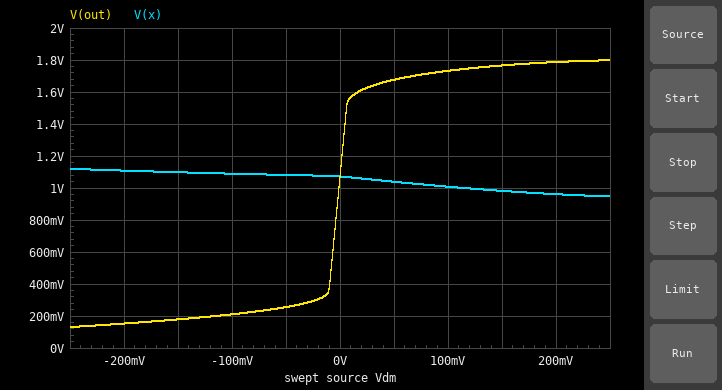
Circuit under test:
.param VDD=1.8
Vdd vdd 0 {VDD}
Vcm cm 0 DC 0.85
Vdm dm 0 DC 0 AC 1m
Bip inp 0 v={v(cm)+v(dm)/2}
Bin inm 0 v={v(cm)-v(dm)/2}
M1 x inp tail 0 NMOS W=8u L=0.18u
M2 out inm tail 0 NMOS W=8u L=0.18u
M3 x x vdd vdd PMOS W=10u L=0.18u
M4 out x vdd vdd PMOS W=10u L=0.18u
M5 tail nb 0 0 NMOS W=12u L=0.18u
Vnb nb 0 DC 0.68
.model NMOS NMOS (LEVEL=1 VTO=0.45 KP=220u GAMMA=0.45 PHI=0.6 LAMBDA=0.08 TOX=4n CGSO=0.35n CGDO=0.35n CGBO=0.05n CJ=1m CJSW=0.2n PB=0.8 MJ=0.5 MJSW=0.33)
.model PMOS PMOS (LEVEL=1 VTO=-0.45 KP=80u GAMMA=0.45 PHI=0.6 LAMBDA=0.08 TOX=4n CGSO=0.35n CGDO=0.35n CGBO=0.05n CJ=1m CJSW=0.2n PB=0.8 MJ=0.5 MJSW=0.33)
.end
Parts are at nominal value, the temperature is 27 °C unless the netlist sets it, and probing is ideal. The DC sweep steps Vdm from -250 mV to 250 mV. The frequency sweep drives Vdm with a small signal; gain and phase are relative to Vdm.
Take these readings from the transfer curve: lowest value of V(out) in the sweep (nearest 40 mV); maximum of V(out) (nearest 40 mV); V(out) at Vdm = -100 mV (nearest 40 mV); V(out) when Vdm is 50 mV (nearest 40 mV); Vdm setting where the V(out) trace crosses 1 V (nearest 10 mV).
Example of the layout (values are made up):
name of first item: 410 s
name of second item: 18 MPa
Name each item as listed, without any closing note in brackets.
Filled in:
lowest value of V(out) in the sweep: 120 mV
maximum of V(out): 1.80 V
V(out) at Vdm = -100 mV: 200 mV
V(out) when Vdm is 50 mV: 1.68 V
Vdm setting where the V(out) trace crosses 1 V: 0 V
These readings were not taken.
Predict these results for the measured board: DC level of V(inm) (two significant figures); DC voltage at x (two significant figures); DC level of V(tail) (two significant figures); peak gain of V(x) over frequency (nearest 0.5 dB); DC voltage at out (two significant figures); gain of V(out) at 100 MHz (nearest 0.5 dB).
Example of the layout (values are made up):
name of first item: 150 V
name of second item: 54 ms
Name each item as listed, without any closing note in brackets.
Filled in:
DC level of V(inm): 850 mV
DC voltage at x: 1.1 V
DC level of V(tail): 170 mV
peak gain of V(x) over frequency: -7.5 dB
DC voltage at out: 1.1 V
gain of V(out) at 100 MHz: 37.0 dB
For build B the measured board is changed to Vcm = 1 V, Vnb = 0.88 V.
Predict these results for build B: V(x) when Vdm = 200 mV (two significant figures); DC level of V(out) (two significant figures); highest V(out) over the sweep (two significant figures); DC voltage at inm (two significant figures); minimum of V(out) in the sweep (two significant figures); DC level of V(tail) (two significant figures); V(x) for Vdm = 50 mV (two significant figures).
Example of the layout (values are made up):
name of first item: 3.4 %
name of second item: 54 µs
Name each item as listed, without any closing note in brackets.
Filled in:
V(x) when Vdm = 200 mV: 780 mV
DC level of V(out): 900 mV
highest V(out) over the sweep: 1.7 V
DC voltage at inm: 1.0 V
minimum of V(out) in the sweep: 210 mV
DC level of V(tail): 190 mV
V(x) for Vdm = 50 mV: 870 mV
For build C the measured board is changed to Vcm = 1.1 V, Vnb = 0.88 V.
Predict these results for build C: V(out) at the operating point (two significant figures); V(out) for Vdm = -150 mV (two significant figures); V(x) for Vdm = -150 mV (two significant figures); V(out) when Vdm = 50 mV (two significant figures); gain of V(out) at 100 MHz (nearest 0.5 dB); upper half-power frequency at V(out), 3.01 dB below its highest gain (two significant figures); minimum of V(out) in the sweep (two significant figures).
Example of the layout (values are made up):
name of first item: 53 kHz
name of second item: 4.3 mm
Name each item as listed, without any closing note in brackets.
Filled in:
V(out) at the operating point: 860 mV
V(out) for Vdm = -150 mV: 340 mV
V(x) for Vdm = -150 mV: 890 mV
V(out) when Vdm = 50 mV: 1.5 V
gain of V(out) at 100 MHz: 32.0 dB
upper half-power frequency at V(out), 3.01 dB below its highest gain: 1.4 GHz
minimum of V(out) in the sweep: 280 mV
